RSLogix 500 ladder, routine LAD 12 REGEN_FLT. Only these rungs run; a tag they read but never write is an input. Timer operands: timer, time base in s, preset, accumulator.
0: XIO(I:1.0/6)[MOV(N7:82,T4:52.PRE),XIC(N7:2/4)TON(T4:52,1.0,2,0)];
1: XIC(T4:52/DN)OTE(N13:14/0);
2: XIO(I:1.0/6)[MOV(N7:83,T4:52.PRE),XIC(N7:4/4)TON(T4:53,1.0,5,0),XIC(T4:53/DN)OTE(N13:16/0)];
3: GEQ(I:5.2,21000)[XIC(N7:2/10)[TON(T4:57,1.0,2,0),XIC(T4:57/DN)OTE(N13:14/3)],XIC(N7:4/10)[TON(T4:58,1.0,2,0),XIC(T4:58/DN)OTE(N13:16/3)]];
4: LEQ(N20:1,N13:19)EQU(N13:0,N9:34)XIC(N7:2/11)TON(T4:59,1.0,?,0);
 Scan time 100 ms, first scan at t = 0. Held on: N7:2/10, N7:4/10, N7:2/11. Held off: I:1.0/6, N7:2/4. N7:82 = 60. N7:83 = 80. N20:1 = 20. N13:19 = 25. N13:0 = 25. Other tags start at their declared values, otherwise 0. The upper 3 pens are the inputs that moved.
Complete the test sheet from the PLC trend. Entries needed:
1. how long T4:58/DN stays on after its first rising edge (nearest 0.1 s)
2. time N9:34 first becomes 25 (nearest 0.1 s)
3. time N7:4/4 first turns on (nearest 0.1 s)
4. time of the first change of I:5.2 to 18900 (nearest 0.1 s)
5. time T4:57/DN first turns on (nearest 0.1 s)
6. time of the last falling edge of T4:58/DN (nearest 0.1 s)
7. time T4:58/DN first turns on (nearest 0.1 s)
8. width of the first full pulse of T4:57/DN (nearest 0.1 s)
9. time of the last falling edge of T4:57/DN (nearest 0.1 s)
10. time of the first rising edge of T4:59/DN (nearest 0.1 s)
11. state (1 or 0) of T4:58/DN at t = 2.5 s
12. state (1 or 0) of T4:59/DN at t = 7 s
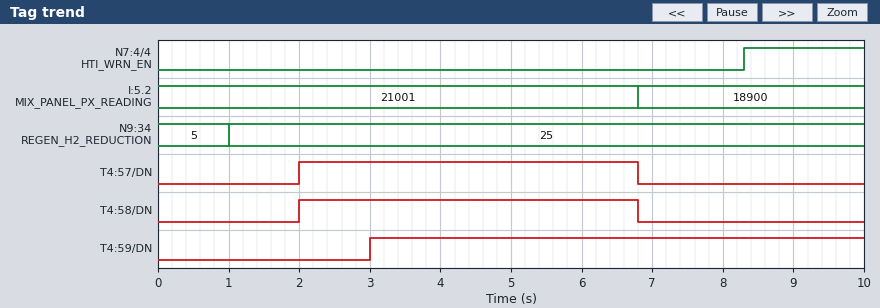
4.8 s
1.0 s
8.3 s
6.8 s
2.0 s
6.8 s
2.0 s
4.8 s
6.8 s
3.0 s
1
1
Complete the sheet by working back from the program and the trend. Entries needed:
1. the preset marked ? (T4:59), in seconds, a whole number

2 s
